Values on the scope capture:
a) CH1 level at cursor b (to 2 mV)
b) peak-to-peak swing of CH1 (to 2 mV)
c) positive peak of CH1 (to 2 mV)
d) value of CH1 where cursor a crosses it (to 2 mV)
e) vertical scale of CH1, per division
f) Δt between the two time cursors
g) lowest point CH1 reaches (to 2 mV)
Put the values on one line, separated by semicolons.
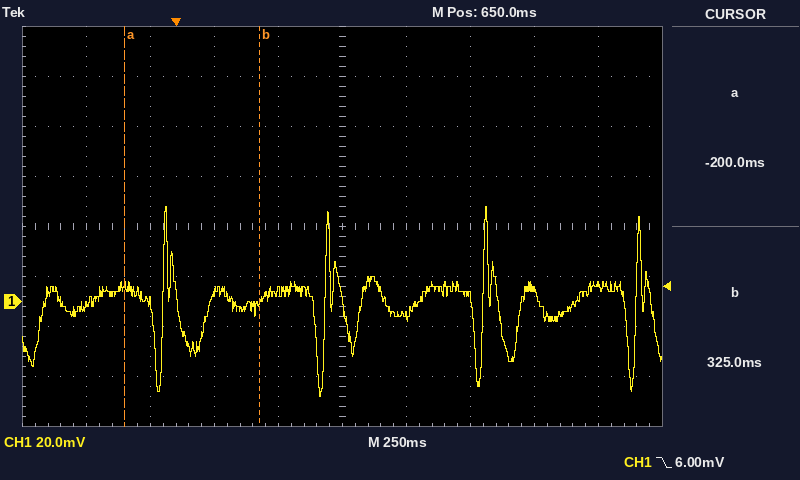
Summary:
0 mV; 76 mV; 38 mV; 6 mV; 20 mV; 525 ms; -38 mV
